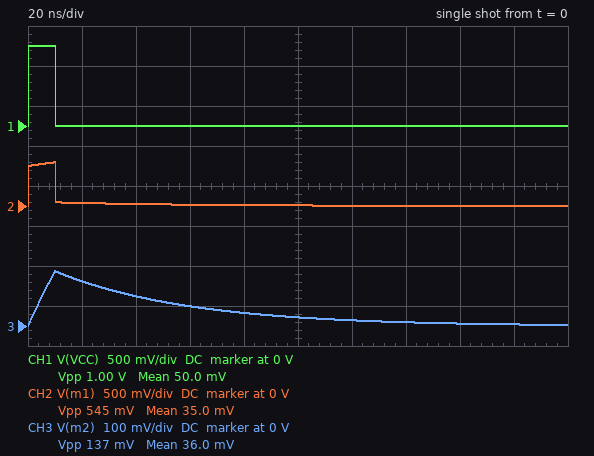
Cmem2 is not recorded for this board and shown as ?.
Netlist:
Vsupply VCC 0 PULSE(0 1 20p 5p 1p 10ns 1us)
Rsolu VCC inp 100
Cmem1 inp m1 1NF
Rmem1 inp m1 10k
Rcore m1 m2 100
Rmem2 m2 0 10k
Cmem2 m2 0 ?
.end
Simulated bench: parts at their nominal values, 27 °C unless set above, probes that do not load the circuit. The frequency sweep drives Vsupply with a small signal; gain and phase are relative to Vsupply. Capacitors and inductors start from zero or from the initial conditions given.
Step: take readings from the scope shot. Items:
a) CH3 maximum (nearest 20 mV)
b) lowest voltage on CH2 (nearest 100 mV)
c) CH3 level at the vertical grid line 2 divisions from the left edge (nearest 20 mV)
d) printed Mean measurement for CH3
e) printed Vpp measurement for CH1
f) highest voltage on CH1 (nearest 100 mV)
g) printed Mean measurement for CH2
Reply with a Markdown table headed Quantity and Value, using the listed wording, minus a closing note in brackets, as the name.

| Quantity | Value |
|---|---|
| CH3 maximum | 140 mV |
| lowest voltage on CH2 | 0 V |
| CH3 level at the vertical grid line 2 divisions from the left edge | 80 mV |
| printed Mean measurement for CH3 | 36.0 mV |
| printed Vpp measurement for CH1 | 1.00 V |
| highest voltage on CH1 | 1.0 V |
| printed Mean measurement for CH2 | 35.0 mV |
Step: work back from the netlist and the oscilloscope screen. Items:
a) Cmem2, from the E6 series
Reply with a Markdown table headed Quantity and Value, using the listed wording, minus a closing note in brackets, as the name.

| Quantity | Value |
|---|---|
| Cmem2, from the E6 series | 330 pF |
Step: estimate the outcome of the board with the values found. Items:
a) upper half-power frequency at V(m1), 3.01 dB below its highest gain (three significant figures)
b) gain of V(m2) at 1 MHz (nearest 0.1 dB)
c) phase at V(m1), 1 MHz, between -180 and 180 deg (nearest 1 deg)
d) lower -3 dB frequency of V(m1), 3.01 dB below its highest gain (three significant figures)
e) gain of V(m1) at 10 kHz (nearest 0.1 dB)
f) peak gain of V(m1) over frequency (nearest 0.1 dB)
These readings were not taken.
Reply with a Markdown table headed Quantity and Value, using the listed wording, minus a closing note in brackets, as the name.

| Quantity | Value |
|---|---|
| upper half-power frequency at V(m1), 3.01 dB below its highest gain | 10.2 MHz |
| gain of V(m2) at 1 MHz | -3.0 dB |
| phase at V(m1), 1 MHz, between -180 and 180 deg | -5 deg |
| lower -3 dB frequency of V(m1), 3.01 dB below its highest gain | 7.63 kHz |
| gain of V(m1) at 10 kHz | -5.3 dB |
| peak gain of V(m1) over frequency | -2.5 dB |
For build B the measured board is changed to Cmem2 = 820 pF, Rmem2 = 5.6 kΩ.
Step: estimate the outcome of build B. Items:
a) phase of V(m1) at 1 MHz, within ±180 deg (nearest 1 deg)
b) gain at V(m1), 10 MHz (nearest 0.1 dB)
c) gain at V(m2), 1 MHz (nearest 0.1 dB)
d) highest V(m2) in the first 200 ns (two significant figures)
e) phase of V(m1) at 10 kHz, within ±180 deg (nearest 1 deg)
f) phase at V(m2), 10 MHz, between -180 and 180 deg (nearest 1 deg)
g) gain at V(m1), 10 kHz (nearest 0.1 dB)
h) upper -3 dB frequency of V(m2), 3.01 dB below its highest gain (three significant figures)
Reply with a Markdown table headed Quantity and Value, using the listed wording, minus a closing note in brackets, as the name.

| Quantity | Value |
|---|---|
| phase of V(m1) at 1 MHz, within ±180 deg | -2 deg |
| gain at V(m1), 10 MHz | -6.0 dB |
| gain at V(m2), 1 MHz | -6.5 dB |
| highest V(m2) in the first 200 ns | 58 mV |
| phase of V(m1) at 10 kHz, within ±180 deg | 10 deg |
| phase at V(m2), 10 MHz, between -180 and 180 deg | -80 deg |
| gain at V(m1), 10 kHz | -8.1 dB |
| upper -3 dB frequency of V(m2), 3.01 dB below its highest gain | 1.83 MHz |
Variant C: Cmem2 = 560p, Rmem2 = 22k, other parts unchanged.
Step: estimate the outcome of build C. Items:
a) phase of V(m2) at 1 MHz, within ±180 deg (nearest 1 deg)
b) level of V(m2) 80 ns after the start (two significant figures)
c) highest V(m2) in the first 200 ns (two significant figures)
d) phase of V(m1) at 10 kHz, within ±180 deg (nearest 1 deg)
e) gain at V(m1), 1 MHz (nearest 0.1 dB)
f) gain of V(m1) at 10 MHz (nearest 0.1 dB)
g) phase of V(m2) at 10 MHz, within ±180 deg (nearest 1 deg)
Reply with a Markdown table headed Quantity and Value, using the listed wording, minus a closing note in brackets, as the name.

| Quantity | Value |
|---|---|
| phase of V(m2) at 1 MHz, within ±180 deg | -24 deg |
| level of V(m2) 80 ns after the start | 31 mV |
| highest V(m2) in the first 200 ns | 83 mV |
| phase of V(m1) at 10 kHz, within ±180 deg | -2 deg |
| gain at V(m1), 1 MHz | -4.2 dB |
| gain of V(m1) at 10 MHz | -5.9 dB |
| phase of V(m2) at 10 MHz, within ±180 deg | -77 deg |
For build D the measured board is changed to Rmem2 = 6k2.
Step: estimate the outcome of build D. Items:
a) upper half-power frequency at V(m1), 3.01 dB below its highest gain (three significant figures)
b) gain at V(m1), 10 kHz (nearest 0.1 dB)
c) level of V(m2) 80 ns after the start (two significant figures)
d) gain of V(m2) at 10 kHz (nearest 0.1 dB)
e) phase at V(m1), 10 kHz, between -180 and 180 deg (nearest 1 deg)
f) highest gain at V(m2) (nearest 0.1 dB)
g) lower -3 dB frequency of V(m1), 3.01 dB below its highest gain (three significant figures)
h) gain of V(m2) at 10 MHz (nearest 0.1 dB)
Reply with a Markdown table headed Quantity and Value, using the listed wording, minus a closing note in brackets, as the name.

| Quantity | Value |
|---|---|
| upper half-power frequency at V(m1), 3.01 dB below its highest gain | 10.5 MHz |
| gain at V(m1), 10 kHz | -7.3 dB |
| level of V(m2) 80 ns after the start | 32 mV |
| gain of V(m2) at 10 kHz | -7.4 dB |
| phase at V(m1), 10 kHz, between -180 and 180 deg | 14 deg |
| highest gain at V(m2) | -2.7 dB |
| lower -3 dB frequency of V(m1), 3.01 dB below its highest gain | 21.0 kHz |
| gain of V(m2) at 10 MHz | -12.8 dB |
